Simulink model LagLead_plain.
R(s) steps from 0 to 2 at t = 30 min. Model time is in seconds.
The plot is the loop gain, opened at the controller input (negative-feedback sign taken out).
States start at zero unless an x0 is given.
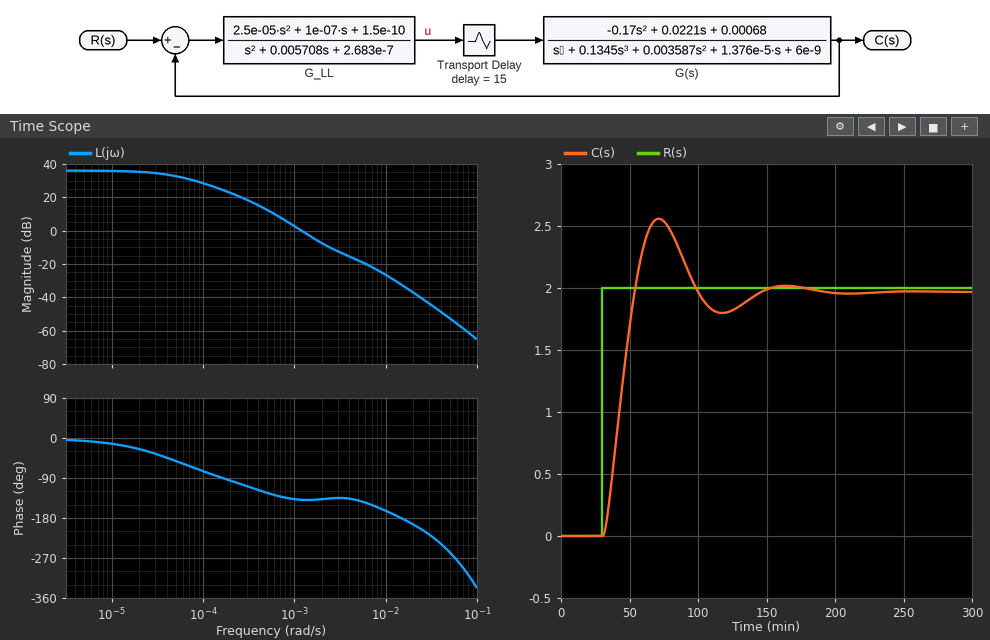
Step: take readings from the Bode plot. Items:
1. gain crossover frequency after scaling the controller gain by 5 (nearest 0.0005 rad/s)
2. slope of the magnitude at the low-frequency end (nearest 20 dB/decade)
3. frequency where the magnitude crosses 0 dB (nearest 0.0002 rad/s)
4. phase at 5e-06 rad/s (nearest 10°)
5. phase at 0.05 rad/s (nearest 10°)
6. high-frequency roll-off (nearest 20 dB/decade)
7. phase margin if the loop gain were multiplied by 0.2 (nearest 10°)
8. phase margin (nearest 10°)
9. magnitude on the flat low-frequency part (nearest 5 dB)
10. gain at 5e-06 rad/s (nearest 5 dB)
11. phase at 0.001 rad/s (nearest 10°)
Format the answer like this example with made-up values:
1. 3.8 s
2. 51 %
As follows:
1. 0.0035 rad/s
2. 0 dB/decade
3. 0.0012 rad/s
4. -10°
5. -260°
6. -40 dB/decade
7. 60°
8. 40°
9. 35 dB
10. 35 dB
11. -140°
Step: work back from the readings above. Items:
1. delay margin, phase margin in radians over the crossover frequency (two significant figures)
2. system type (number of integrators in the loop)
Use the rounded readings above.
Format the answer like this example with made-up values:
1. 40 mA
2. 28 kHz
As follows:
1. 580 s
2. 0
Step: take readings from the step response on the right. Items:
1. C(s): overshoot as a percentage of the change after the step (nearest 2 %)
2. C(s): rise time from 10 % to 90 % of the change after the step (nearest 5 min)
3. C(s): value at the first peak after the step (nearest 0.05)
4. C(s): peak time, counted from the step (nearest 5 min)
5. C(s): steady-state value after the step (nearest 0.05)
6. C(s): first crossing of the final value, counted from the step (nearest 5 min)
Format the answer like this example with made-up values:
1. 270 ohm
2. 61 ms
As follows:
1. 30 %
2. 15 min
3. 2.55
4. 40 min
5. 1.95
6. 25 min
